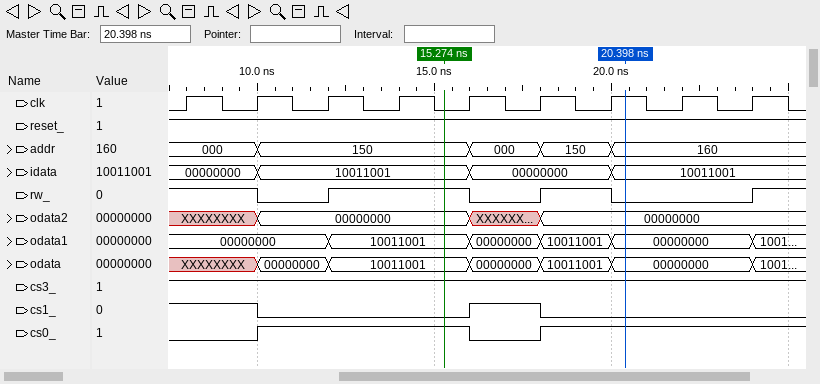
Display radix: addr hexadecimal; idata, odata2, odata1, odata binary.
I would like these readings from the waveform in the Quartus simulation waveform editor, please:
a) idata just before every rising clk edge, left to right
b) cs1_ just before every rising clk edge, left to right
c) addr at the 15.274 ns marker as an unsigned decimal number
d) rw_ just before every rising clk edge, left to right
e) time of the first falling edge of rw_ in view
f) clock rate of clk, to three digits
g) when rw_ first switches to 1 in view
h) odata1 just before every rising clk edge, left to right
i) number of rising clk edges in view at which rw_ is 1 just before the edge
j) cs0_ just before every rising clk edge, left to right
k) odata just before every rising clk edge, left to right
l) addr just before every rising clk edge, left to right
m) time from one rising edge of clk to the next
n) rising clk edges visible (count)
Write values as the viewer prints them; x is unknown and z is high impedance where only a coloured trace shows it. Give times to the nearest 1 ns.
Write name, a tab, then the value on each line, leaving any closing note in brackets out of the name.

idata just before every rising clk edge, left to right	00000000, 00000000, 10011001, 10011001, 10011001, 00000000, 00000000, 10011001, 10011001
cs1_ just before every rising clk edge, left to right	1 1 0 0 0 1 0 0 0
addr at the 15.274 ns marker as an unsigned decimal number	336
rw_ just before every rising clk edge, left to right	1 1 0 1 1 0 1 0 0
time of the first falling edge of rw_ in view	10 ns
clock rate of clk, to three digits	500 MHz
when rw_ first switches to 1 in view	12 ns
odata1 just before every rising clk edge, left to right	00000000, 00000000, 00000000, 10011001, 10011001, 00000000, 10011001, 00000000, 00000000
number of rising clk edges in view at which rw_ is 1 just before the edge	5
cs0_ just before every rising clk edge, left to right	0 0 1 1 1 0 1 1 1
odata just before every rising clk edge, left to right	XXXXXXXX, XXXXXXXX, 00000000, 10011001, 10011001, 00000000, 10011001, 00000000, 00000000
addr just before every rising clk edge, left to right	000, 000, 150, 150, 150, 000, 150, 160, 160
time from one rising edge of clk to the next	2 ns
rising clk edges visible	9
